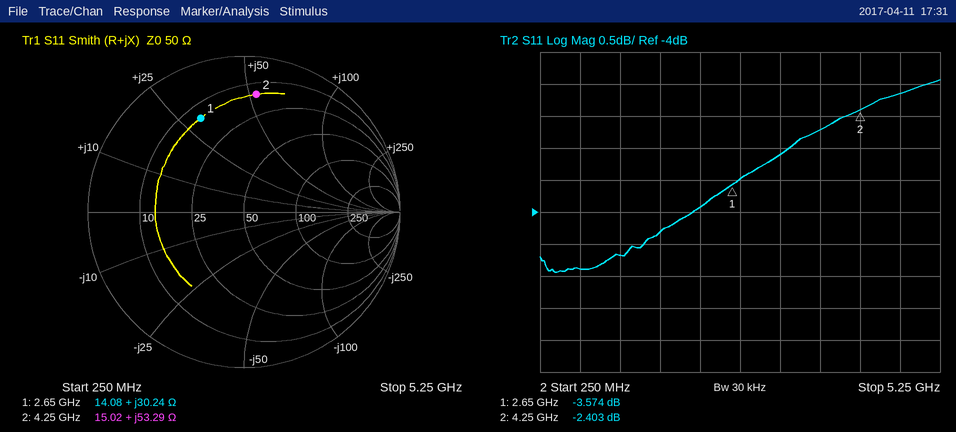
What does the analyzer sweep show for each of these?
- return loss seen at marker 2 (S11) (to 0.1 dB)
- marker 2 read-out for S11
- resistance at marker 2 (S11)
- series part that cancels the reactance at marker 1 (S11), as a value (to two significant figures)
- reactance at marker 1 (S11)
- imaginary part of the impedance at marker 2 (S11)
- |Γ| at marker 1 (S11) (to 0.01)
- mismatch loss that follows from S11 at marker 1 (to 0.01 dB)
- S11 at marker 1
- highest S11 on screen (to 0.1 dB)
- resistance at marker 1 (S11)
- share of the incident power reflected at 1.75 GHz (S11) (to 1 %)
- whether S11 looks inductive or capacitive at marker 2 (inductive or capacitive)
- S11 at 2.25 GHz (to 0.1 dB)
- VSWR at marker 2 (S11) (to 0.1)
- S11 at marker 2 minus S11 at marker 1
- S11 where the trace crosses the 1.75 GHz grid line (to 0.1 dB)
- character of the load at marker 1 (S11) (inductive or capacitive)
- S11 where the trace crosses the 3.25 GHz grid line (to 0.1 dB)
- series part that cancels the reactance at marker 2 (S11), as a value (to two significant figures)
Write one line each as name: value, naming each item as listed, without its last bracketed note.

return loss seen at marker 2 (S11): 2.4 dB
marker 2 read-out for S11: -2.403 dB
resistance at marker 2: 15.02 Ω
series part that cancels the reactance at marker 1 (S11), as a value: 2.0 pF
reactance at marker 1: +30.24 Ω
imaginary part of the impedance at marker 2: +53.29 Ω
|Γ| at marker 1 (S11): 0.66
mismatch loss that follows from S11 at marker 1: 2.51 dB
S11 at marker 1: -3.574 dB
highest S11 on screen: -1.9 dB
resistance at marker 1: 14.08 Ω
share of the incident power reflected at 1.75 GHz (S11): 37 %
whether S11 looks inductive or capacitive at marker 2: inductive
S11 at 2.25 GHz: -3.9 dB
VSWR at marker 2 (S11): 7.3
S11 at marker 2 minus S11 at marker 1: 1.171 dB
S11 where the trace crosses the 1.75 GHz grid line: -4.3 dB
character of the load at marker 1 (S11): inductive
S11 where the trace crosses the 3.25 GHz grid line: -3.1 dB
series part that cancels the reactance at marker 2 (S11), as a value: 700 fF
